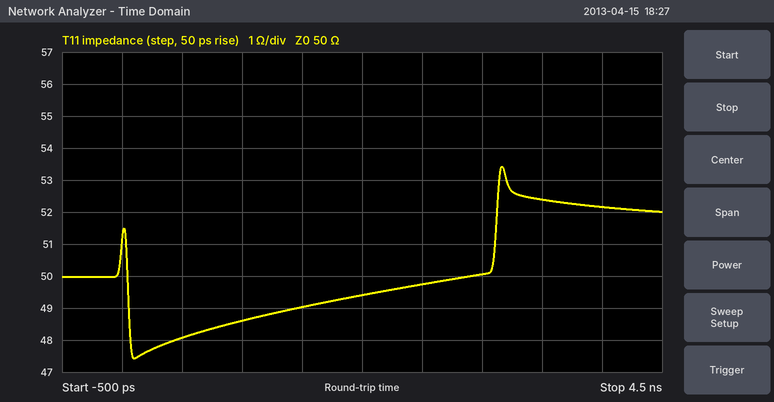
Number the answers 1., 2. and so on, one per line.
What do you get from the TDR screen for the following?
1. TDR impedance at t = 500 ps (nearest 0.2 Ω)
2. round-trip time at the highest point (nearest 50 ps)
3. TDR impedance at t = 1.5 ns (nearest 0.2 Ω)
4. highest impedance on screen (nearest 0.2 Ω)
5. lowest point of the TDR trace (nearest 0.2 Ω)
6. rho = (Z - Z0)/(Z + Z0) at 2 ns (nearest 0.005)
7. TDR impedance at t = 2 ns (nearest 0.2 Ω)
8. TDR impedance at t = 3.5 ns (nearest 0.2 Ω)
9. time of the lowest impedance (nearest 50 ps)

1. 48.0 Ω
2. 3.15 ns
3. 49.0 Ω
4. 53.4 Ω
5. 47.4 Ω
6. -0.005
7. 49.4 Ω
8. 52.4 Ω
9. 100 ps
